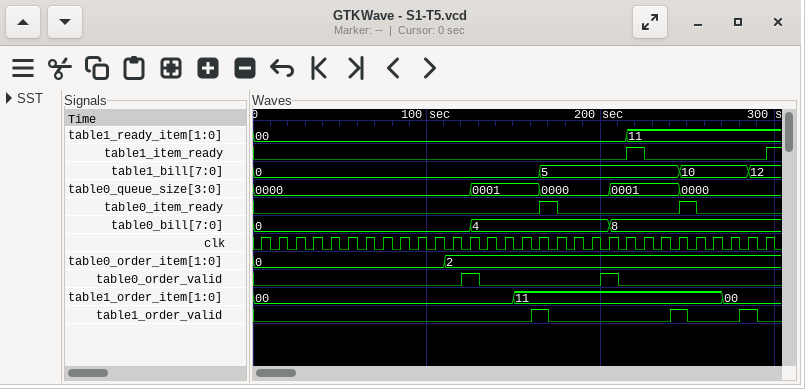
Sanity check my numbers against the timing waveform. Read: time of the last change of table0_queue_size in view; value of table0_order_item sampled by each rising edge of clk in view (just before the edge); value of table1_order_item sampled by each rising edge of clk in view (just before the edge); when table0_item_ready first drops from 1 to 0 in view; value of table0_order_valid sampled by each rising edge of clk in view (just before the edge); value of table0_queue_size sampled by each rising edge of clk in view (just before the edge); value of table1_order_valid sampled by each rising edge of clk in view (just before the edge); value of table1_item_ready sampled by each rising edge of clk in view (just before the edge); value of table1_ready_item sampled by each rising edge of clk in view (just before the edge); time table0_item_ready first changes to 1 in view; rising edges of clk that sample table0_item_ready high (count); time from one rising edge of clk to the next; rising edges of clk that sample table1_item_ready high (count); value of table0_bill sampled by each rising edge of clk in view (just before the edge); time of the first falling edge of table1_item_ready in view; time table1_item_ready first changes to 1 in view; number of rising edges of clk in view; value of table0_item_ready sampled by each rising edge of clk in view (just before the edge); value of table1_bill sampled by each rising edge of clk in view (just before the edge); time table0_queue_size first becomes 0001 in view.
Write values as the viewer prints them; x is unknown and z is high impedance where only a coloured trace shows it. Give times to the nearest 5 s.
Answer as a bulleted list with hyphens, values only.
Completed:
- 245 s
- 0, 0, 0, 0, 0, 0, 0, 0, 0, 0, 0, 2, 2, 2, 2, 2, 2, 2, 2, 2, 2, 2, 2, 2, 2, 2, 2, 2, 2, 2
- 00, 00, 00, 00, 00, 00, 00, 00, 00, 00, 00, 00, 00, 00, 00, 11, 11, 11, 11, 11, 11, 11, 11, 11, 11, 11, 11, 00, 00, 00
- 175 s
- 0 0 0 0 0 0 0 0 0 0 0 0 1 0 0 0 0 0 0 0 1 0 0 0 0 0 0 0 0 0
- 0000, 0000, 0000, 0000, 0000, 0000, 0000, 0000, 0000, 0000, 0000, 0000, 0000, 0001, 0001, 0001, 0001, 0000, 0000, 0000, 0000, 0001, 0001, 0001, 0001, 0000, 0000, 0000, 0000, 0000
- 0 0 0 0 0 0 0 0 0 0 0 0 0 0 0 0 1 0 0 0 0 0 0 0 1 0 0 0 1 0
- 0 0 0 0 0 0 0 0 0 0 0 0 0 0 0 0 0 0 0 0 0 0 1 0 0 0 0 0 0 0
- 00, 00, 00, 00, 00, 00, 00, 00, 00, 00, 00, 00, 00, 00, 00, 00, 00, 00, 00, 00, 00, 00, 11, 11, 11, 11, 11, 11, 11, 11
- 165 s
- 2
- 10 s
- 1
- 0, 0, 0, 0, 0, 0, 0, 0, 0, 0, 0, 0, 0, 4, 4, 4, 4, 4, 4, 4, 4, 8, 8, 8, 8, 8, 8, 8, 8, 8
- 225 s
- 215 s
- 30
- 0 0 0 0 0 0 0 0 0 0 0 0 0 0 0 0 0 1 0 0 0 0 0 0 0 1 0 0 0 0
- 0, 0, 0, 0, 0, 0, 0, 0, 0, 0, 0, 0, 0, 0, 0, 0, 0, 5, 5, 5, 5, 5, 5, 5, 5, 10, 10, 10, 10, 12
- 125 s
